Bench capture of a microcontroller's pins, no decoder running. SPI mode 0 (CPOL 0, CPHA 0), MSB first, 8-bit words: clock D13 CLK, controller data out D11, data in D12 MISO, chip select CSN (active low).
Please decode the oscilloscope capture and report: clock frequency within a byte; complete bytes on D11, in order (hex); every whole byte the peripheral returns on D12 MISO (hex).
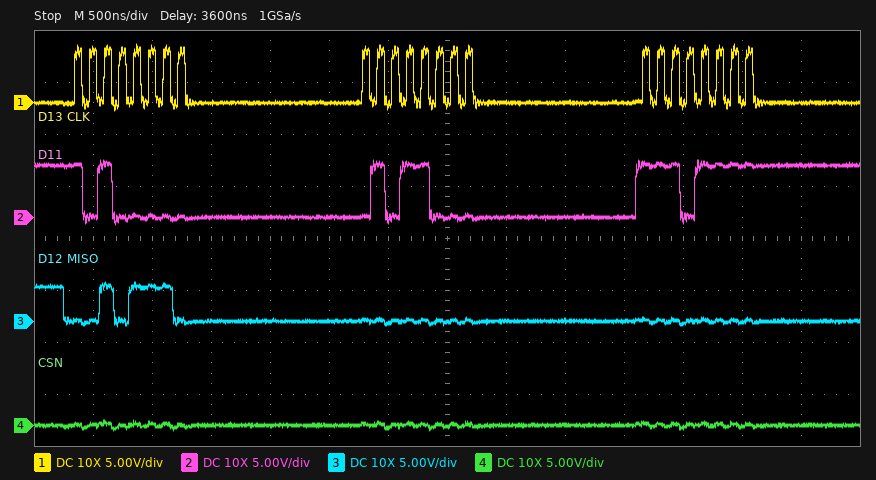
8 MHz
A0 58 EF
2E 00 00
